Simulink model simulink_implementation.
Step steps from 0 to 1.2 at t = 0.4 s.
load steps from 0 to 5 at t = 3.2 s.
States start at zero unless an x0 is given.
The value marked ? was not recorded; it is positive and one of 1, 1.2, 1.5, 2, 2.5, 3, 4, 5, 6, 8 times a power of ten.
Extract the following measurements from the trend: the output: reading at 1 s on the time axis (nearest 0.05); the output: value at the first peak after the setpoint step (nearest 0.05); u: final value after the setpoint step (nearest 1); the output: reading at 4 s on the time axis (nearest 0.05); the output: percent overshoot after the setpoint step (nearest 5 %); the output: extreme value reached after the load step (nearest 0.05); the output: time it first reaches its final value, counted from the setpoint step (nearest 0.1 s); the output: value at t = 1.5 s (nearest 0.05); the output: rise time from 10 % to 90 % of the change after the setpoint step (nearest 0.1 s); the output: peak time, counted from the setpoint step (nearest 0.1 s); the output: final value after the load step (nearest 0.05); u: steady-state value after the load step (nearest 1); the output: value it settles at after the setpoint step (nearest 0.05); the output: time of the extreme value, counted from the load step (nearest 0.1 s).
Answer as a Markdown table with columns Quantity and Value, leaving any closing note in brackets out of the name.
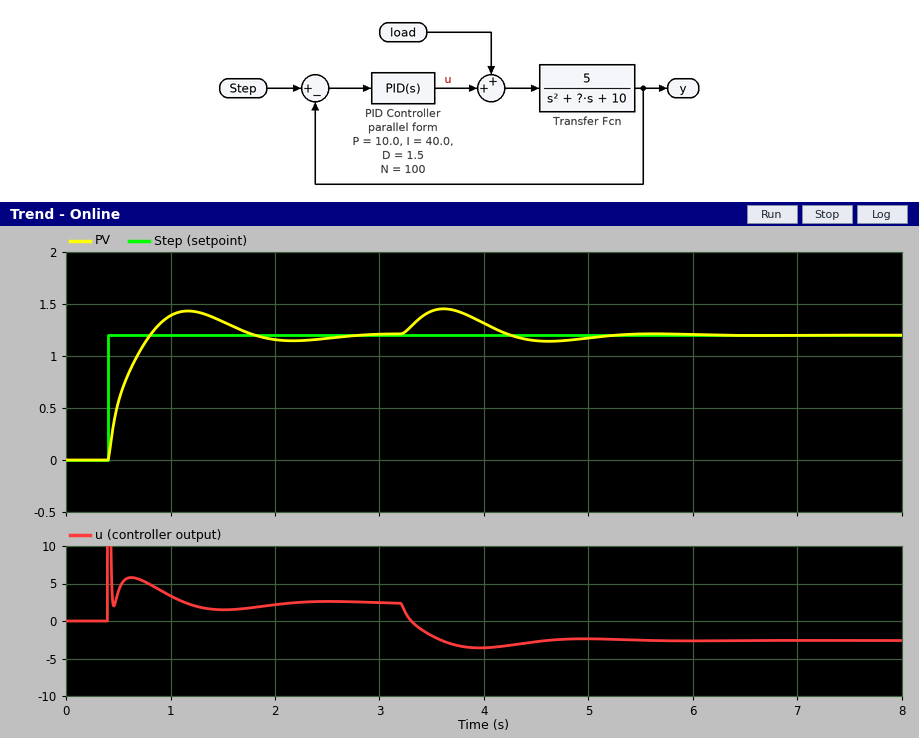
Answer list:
| Quantity | Value |
|---|---|
| the output: reading at 1 s on the time axis | 1.40 |
| the output: value at the first peak after the setpoint step | 1.45 |
| u: final value after the setpoint step | 2 |
| the output: reading at 4 s on the time axis | 1.30 |
| the output: percent overshoot after the setpoint step | 20 % |
| the output: extreme value reached after the load step | 1.45 |
| the output: time it first reaches its final value, counted from the setpoint step | 0.4 s |
| the output: value at t = 1.5 s | 1.35 |
| the output: rise time from 10 % to 90 % of the change after the setpoint step | 0.3 s |
| the output: peak time, counted from the setpoint step | 0.8 s |
| the output: final value after the load step | 1.20 |
| u: steady-state value after the load step | -3 |
| the output: value it settles at after the setpoint step | 1.20 |
| the output: time of the extreme value, counted from the load step | 0.4 s |
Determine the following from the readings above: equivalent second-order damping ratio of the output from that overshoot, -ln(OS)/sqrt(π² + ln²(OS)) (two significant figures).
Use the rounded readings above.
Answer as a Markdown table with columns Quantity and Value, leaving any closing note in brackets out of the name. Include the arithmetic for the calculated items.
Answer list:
| Quantity | Value |
|---|---|
| equivalent second-order damping ratio of the output from that overshoot, -ln(OS)/sqrt(π² + ln²(OS)) | ln(0.2) = -1.609; 1.609 / sqrt(9.870 + 2.590) = 0.46 |
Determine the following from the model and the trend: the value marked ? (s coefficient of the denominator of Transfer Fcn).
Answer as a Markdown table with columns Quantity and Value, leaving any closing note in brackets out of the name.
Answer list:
| Quantity | Value |
|---|---|
| the value marked ? | 12 |
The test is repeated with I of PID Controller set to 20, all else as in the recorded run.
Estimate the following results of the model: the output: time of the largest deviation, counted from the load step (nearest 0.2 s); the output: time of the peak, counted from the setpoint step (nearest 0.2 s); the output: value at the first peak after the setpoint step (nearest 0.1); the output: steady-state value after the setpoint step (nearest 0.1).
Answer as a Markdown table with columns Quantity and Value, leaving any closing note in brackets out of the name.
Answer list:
| Quantity | Value |
|---|---|
| the output: time of the largest deviation, counted from the load step | 0.6 s |
| the output: time of the peak, counted from the setpoint step | 1.0 s |
| the output: value at the first peak after the setpoint step | 1.3 |
| the output: steady-state value after the setpoint step | 1.2 |
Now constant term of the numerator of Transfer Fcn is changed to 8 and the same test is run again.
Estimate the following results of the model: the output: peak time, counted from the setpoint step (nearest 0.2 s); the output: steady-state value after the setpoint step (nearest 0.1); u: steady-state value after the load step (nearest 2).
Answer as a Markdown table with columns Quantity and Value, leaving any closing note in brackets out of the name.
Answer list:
| Quantity | Value |
|---|---|
| the output: peak time, counted from the setpoint step | 0.6 s |
| the output: steady-state value after the setpoint step | 1.2 |
| u: steady-state value after the load step | -4 |
